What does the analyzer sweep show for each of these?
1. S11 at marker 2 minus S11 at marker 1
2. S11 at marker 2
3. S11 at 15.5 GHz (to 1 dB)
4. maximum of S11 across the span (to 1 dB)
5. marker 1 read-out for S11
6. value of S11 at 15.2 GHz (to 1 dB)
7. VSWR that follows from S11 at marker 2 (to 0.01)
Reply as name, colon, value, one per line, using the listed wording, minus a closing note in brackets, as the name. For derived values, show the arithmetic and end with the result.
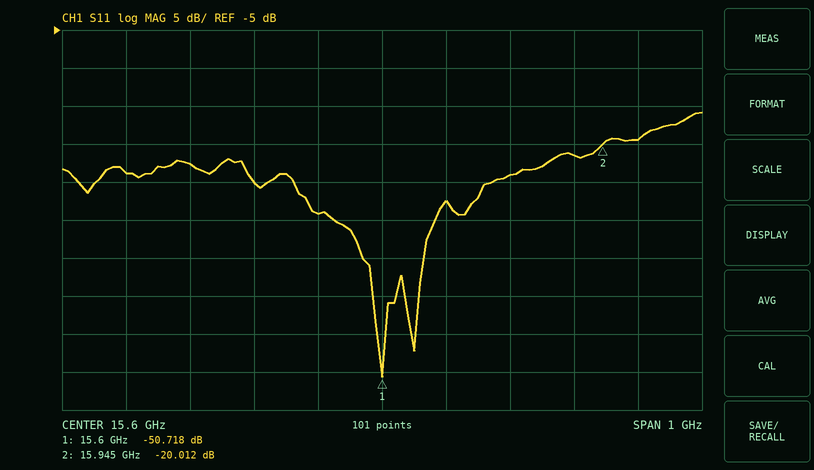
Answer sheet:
S11 at marker 2 minus S11 at marker 1: -20.012 − (-50.718) = 30.706 dB
S11 at marker 2: -20.012 dB
S11 at 15.5 GHz: -29 dB
maximum of S11 across the span: -16 dB
marker 1 read-out for S11: -50.718 dB
value of S11 at 15.2 GHz: -24 dB
VSWR that follows from S11 at marker 2: (1 + 0.0999)/(1 − 0.0999) ≈ 1.22
